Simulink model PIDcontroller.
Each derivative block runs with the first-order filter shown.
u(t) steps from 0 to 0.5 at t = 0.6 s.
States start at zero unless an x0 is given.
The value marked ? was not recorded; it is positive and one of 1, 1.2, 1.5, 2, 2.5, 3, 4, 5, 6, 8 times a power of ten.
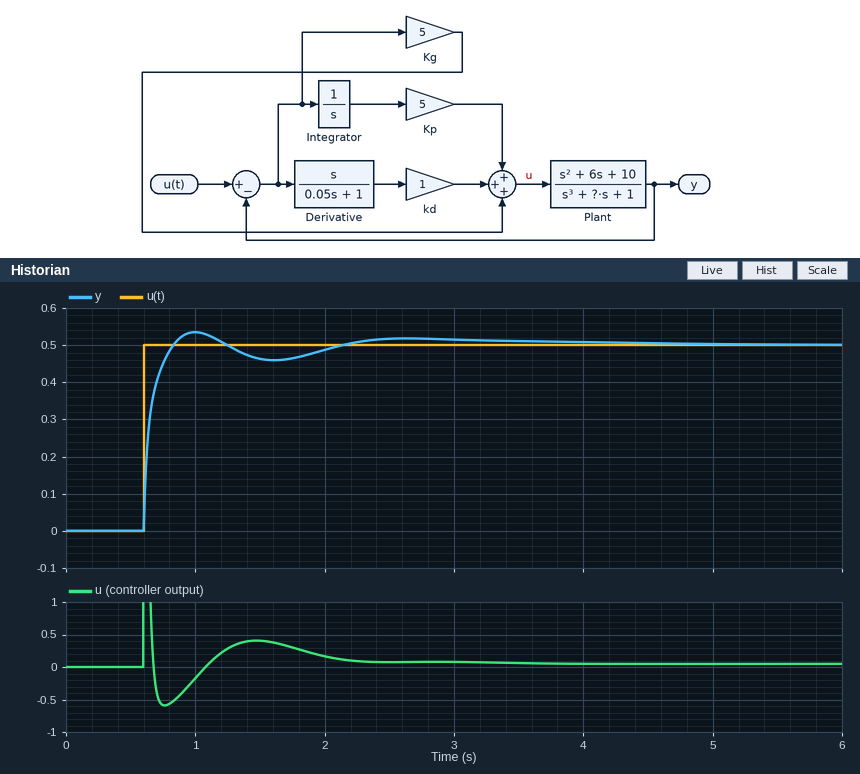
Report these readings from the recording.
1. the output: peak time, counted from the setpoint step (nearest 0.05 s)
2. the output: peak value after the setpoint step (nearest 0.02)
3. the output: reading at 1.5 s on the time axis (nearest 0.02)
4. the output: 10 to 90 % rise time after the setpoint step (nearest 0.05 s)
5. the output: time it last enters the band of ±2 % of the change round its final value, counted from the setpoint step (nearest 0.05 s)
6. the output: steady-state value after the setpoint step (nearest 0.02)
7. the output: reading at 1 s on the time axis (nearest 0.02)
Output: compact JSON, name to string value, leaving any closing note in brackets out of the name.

{"the output: peak time, counted from the setpoint step": "0.40 s", "the output: peak value after the setpoint step": "0.54", "the output: reading at 1.5 s on the time axis": "0.46", "the output: 10 to 90 % rise time after the setpoint step": "0.15 s", "the output: time it last enters the band of ±2 % of the change round its final value, counted from the setpoint step": "3.10 s", "the output: steady-state value after the setpoint step": "0.50", "the output: reading at 1 s on the time axis": "0.54"}
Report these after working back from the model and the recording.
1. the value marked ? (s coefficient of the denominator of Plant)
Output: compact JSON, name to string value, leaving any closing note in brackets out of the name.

{"the value marked ?": "8"}
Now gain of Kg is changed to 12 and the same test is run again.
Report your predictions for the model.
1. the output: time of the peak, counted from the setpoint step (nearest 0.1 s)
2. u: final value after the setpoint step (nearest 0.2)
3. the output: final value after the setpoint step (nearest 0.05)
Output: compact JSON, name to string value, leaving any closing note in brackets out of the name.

{"the output: time of the peak, counted from the setpoint step": "0.3 s", "u: final value after the setpoint step": "0.0", "the output: final value after the setpoint step": "0.50"}
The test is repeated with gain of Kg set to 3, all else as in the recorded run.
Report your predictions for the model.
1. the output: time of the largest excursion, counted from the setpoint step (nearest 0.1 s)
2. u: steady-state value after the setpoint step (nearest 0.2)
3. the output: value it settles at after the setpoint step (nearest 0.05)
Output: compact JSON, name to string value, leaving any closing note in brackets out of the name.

{"the output: time of the largest excursion, counted from the setpoint step": "2.1 s", "u: steady-state value after the setpoint step": "0.0", "the output: value it settles at after the setpoint step": "0.50"}
